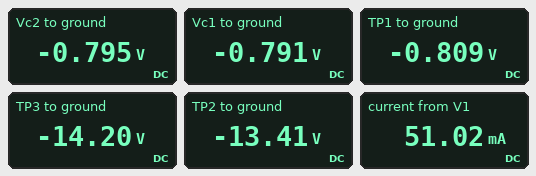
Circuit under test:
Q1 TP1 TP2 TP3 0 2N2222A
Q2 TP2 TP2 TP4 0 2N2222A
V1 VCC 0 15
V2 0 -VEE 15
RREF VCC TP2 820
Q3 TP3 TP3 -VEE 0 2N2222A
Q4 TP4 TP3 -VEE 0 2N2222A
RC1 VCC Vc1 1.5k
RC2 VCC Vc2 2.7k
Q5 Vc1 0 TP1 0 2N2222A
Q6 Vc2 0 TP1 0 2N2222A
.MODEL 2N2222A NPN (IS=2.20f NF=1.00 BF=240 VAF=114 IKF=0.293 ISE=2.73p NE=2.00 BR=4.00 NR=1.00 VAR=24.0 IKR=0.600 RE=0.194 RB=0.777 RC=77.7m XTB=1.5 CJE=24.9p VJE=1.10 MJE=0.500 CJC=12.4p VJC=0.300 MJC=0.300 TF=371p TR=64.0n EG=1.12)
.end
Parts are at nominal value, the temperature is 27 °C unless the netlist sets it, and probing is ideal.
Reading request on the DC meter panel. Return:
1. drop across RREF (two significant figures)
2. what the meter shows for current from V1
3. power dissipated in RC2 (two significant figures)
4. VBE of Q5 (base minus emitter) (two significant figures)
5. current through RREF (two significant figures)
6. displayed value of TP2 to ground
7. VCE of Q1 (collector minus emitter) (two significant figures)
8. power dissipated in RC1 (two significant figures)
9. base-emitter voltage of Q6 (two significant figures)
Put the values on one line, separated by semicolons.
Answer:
28 V; 51.02 mA; 92 mW; 810 mV; 35 mA; -13.41 V; 13 V; 170 mW; 810 mV
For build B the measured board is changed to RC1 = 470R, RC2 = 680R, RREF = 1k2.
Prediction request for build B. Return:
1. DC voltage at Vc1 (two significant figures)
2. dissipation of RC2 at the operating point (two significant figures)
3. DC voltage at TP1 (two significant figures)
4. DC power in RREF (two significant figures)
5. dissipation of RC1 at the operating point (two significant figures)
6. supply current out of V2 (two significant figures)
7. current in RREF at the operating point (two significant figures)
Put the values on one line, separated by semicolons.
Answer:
9.4 V; 93 mW; -760 mV; 670 mW; 67 mW; 47 mA; 24 mA
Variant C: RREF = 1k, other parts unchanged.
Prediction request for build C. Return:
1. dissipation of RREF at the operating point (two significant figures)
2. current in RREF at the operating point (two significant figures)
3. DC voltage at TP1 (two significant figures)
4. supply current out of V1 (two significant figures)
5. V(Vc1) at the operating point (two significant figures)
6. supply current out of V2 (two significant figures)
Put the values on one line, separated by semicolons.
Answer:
810 mW; 28 mA; -800 mV; 45 mA; -780 mV; 57 mA
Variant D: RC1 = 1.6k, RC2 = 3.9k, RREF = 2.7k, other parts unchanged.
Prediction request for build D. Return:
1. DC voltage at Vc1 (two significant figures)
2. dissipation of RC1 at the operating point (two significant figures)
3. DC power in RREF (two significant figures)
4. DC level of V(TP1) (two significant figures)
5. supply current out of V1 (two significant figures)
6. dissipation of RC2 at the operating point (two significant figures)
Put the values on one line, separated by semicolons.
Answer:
5.2 V; 60 mW; 300 mW; -740 mV; 21 mA; 63 mW
